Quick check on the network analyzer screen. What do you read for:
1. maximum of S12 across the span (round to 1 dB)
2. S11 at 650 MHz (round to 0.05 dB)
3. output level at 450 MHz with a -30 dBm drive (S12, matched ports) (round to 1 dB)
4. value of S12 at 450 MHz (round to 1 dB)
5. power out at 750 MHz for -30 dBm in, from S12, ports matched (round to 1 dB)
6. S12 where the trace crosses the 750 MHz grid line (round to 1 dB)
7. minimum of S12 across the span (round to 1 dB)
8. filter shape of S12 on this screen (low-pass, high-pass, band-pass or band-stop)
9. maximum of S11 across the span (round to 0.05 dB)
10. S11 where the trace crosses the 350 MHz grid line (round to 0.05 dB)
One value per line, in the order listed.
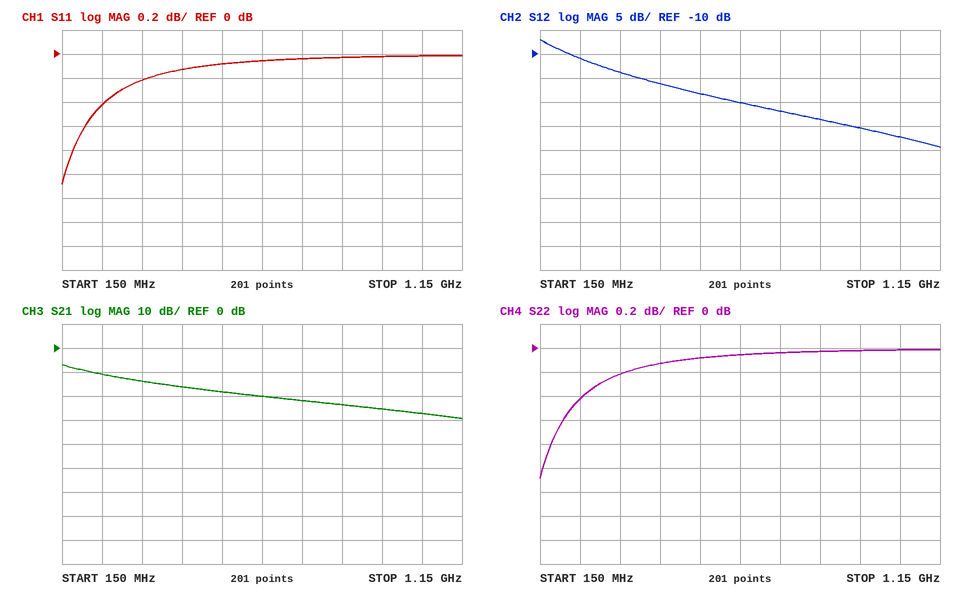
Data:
-7 dB
-0.05 dB
-46 dBm
-16 dB
-52 dBm
-22 dB
-29 dB
low-pass
0.00 dB
-0.20 dB
